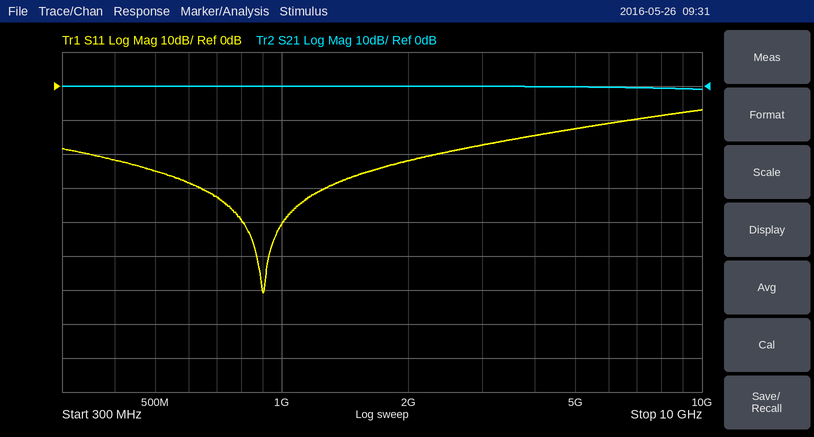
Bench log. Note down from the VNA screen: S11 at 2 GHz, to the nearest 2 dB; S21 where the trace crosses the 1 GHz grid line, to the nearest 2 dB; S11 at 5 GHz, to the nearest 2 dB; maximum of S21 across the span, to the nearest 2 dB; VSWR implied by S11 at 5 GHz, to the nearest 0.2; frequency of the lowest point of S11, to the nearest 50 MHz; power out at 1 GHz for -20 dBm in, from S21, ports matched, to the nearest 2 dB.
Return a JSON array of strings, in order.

["-22 dB", "0 dB", "-12 dB", "0 dB", "1.6", "900 MHz", "-20 dBm"]
